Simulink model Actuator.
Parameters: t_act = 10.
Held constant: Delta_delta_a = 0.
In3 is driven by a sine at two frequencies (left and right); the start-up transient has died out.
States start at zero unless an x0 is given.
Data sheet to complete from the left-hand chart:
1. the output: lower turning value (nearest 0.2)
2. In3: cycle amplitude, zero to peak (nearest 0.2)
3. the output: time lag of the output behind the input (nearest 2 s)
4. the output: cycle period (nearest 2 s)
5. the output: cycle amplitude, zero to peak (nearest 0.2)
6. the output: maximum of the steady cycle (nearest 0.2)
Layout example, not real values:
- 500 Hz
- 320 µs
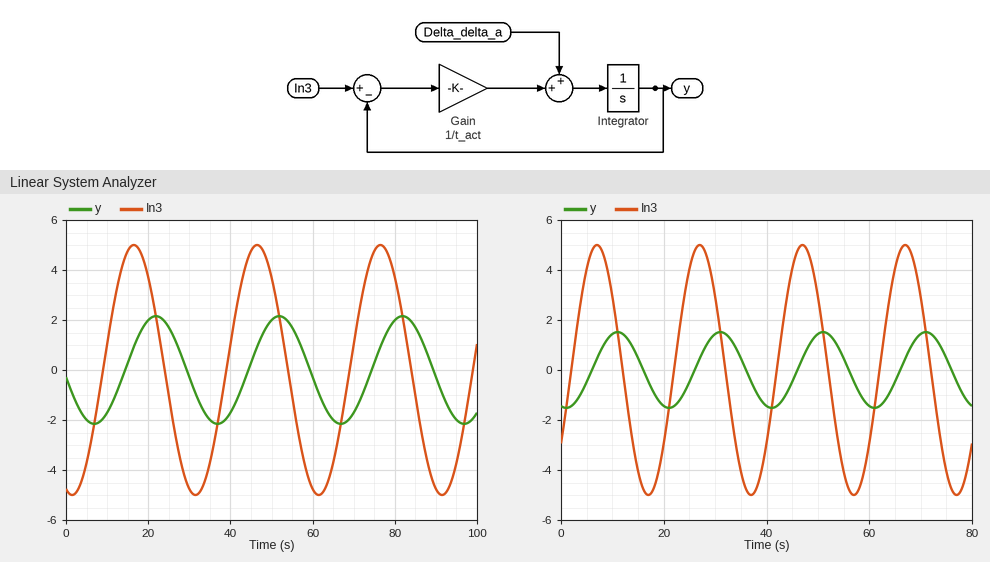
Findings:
- -2.2
- 5.0
- 6 s
- 30 s
- 2.2
- 2.2
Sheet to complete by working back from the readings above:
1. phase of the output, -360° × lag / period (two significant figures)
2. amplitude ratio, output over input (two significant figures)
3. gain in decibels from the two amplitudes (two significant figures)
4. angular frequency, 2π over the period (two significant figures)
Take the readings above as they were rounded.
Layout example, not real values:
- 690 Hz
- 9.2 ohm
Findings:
- -72°
- 0.44
- -7.1 dB
- 0.21 rad/s
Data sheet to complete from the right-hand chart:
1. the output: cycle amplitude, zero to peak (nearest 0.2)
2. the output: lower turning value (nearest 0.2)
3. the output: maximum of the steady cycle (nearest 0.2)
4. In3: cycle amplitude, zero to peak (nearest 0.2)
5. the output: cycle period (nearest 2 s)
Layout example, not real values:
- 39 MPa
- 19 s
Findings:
- 1.6
- -1.6
- 1.6
- 5.0
- 20 s
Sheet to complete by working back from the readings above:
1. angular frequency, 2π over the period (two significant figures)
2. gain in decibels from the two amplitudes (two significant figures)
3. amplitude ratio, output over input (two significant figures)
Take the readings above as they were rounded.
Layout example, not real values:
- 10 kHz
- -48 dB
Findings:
- 0.31 rad/s
- -9.9 dB
- 0.32
